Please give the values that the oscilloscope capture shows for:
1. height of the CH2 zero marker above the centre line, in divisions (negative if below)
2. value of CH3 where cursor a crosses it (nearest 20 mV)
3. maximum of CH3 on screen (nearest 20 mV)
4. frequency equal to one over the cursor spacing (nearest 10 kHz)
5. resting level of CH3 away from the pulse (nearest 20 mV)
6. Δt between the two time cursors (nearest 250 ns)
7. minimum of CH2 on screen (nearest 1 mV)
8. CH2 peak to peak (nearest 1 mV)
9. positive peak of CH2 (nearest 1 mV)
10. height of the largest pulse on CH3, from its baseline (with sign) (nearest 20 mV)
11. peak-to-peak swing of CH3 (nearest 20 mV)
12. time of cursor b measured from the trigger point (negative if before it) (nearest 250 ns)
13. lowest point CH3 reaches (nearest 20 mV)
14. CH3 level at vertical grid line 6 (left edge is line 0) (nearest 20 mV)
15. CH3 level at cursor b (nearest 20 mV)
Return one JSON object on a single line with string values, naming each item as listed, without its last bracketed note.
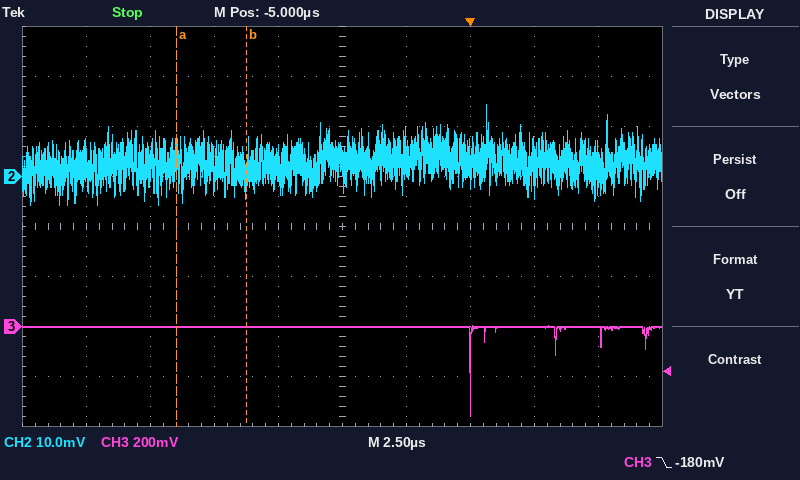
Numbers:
{"height of the CH2 zero marker above the centre line, in divisions": "+1.0 div", "value of CH3 where cursor a crosses it": "0 mV", "maximum of CH3 on screen": "0 mV", "frequency equal to one over the cursor spacing": "360 kHz", "resting level of CH3 away from the pulse": "0 mV", "Δt between the two time cursors": "2.75 µs", "minimum of CH2 on screen": "-6 mV", "CH2 peak to peak": "20 mV", "positive peak of CH2": "14 mV", "height of the largest pulse on CH3, from its baseline (with sign)": "-360 mV", "peak-to-peak swing of CH3": "360 mV", "time of cursor b measured from the trigger point (negative if before it)": "-8.75 µs", "lowest point CH3 reaches": "-360 mV", "CH3 level at vertical grid line 6 (left edge is line 0)": "0 mV", "CH3 level at cursor b": "0 mV"}
